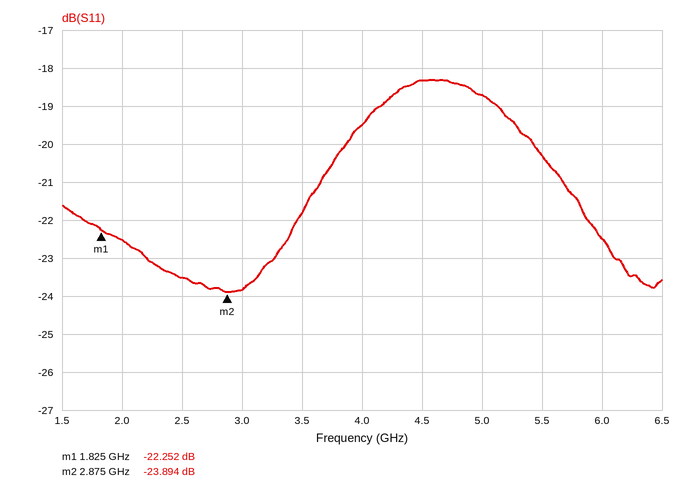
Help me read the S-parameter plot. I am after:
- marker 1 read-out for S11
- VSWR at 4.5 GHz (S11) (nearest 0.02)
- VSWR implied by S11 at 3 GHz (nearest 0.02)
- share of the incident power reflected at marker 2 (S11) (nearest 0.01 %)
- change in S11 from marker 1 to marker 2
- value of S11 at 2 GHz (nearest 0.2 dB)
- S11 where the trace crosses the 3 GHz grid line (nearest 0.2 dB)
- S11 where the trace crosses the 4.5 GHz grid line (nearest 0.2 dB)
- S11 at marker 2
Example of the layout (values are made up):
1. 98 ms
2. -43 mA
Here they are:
1. -22.252 dB
2. 1.28
3. 1.14
4. 0.41 %
5. -1.642 dB
6. -22.6 dB
7. -23.8 dB
8. -18.4 dB
9. -23.894 dB
